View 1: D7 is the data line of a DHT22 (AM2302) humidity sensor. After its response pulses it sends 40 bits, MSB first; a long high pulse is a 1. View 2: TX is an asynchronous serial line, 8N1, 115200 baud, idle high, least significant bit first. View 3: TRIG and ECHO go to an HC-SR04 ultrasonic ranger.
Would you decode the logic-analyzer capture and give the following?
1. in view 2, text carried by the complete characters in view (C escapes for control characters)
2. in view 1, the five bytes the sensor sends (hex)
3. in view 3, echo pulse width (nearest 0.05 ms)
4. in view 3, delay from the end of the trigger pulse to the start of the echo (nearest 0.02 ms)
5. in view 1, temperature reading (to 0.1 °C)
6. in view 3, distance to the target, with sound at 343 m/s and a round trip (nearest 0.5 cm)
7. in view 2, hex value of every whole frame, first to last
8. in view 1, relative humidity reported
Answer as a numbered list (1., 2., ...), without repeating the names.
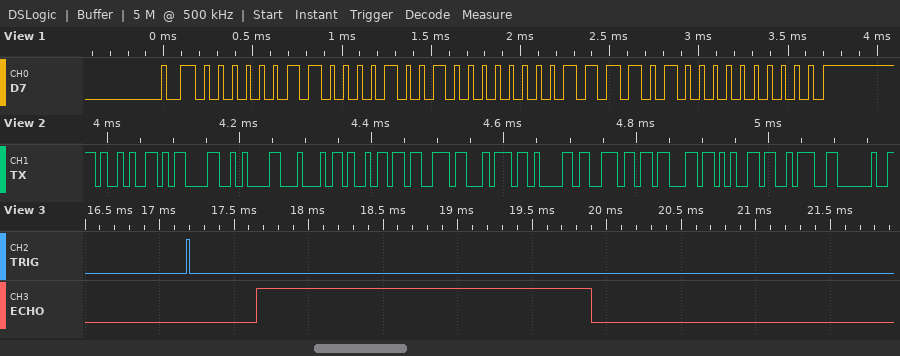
1. ")\r\nDistance: "
2. 03 09 00 F4 00
3. 2.25 ms
4. 0.46 ms
5. 24.4 °C
6. 38.5 cm
7. 29 0D 0A 44 69 73 74 61 6E 63 65 3A 20
8. 77.7 %
